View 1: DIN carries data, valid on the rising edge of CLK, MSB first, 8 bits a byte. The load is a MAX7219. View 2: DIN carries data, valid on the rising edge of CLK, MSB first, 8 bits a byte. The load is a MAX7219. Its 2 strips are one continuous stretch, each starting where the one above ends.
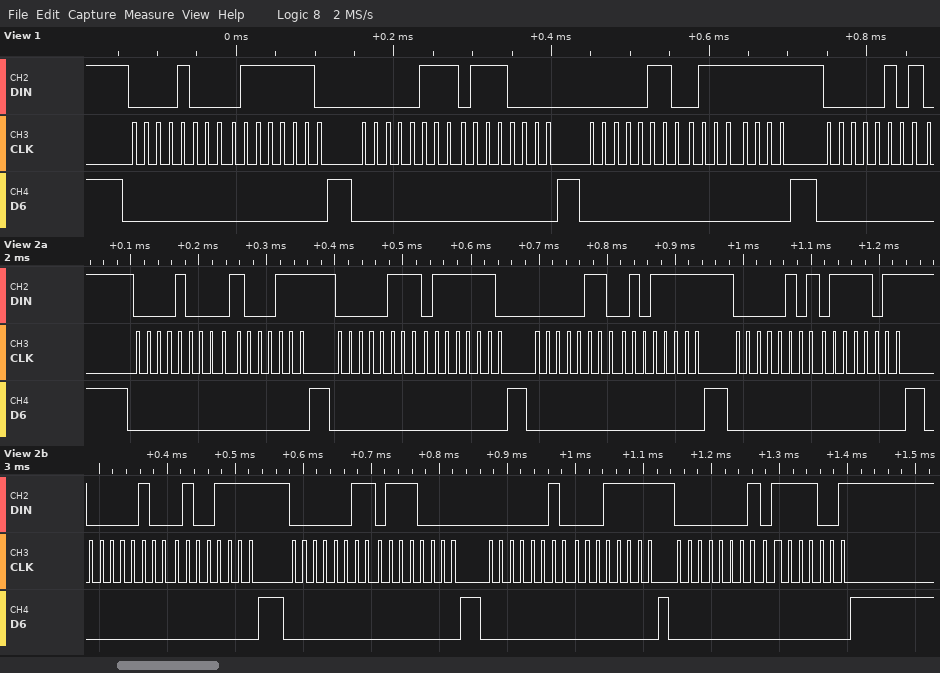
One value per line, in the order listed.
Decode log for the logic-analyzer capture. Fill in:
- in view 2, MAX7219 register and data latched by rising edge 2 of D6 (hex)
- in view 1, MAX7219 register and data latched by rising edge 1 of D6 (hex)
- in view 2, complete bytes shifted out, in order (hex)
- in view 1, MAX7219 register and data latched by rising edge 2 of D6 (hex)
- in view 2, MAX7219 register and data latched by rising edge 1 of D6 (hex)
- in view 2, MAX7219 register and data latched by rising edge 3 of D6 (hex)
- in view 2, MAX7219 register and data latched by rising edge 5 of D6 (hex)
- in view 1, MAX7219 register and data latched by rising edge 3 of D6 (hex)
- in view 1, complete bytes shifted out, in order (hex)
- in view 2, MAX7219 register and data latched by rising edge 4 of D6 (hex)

register 0x7, data 0x7E
register 0x8, data 0x7E
0x08 0x47 0x07 0x7E 0x06 0x5F 0x05 0x7B 0x04 0x4F 0x03 0x70 0x02 0x1F 0x01 0x79
register 0x7, data 0x70
register 0x8, data 0x47
register 0x6, data 0x5F
register 0x4, data 0x4F
register 0x6, data 0x7F
08 7E 07 70 06 7F 05
register 0x5, data 0x7B
